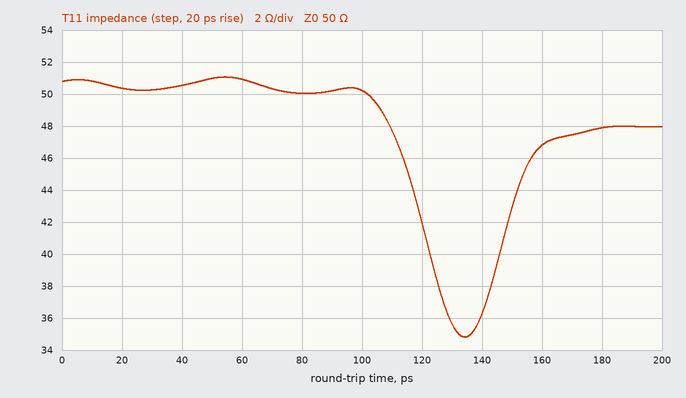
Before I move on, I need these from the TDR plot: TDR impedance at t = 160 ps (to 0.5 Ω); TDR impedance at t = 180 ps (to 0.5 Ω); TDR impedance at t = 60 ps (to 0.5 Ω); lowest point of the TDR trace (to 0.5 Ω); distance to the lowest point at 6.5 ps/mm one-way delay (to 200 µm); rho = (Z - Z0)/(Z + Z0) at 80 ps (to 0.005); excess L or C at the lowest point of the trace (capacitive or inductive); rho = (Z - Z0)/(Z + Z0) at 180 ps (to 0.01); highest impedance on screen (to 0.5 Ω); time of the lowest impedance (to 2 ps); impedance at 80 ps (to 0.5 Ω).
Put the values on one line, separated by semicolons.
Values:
47.0 Ω; 48.0 Ω; 51.0 Ω; 35.0 Ω; 10.4 mm; 0.000; capacitive; -0.02; 51.0 Ω; 134 ps; 50.0 Ω
